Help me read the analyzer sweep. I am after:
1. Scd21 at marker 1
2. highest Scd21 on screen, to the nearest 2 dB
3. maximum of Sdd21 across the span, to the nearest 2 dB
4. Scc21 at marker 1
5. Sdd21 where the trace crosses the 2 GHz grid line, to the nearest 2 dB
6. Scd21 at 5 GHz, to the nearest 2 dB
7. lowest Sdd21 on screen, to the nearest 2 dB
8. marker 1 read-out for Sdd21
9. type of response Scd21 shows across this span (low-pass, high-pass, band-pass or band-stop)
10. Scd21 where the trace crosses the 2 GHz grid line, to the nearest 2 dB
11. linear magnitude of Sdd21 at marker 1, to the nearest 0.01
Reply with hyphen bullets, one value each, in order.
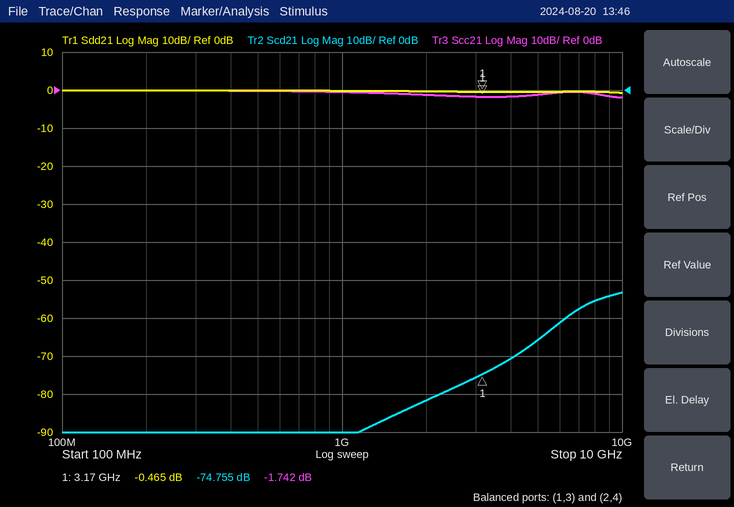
- -74.755 dB
- -54 dB
- 0 dB
- -1.742 dB
- 0 dB
- -66 dB
- 0 dB
- -0.465 dB
- high-pass
- -82 dB
- 0.95
